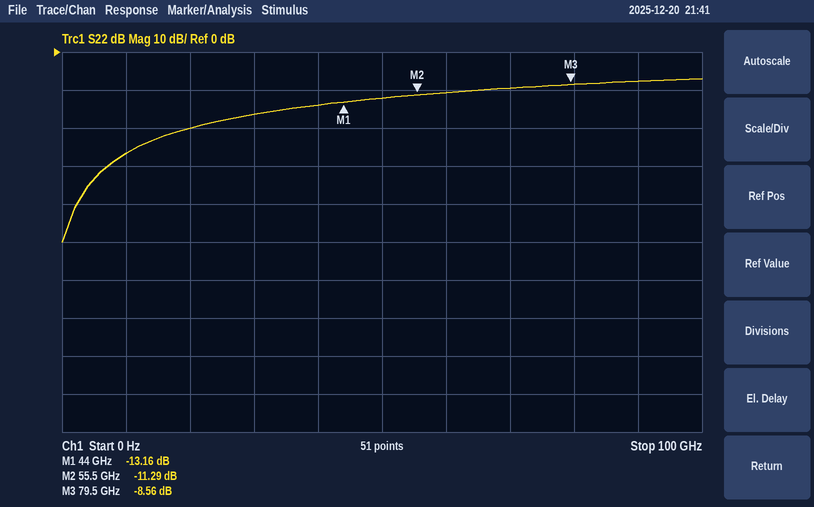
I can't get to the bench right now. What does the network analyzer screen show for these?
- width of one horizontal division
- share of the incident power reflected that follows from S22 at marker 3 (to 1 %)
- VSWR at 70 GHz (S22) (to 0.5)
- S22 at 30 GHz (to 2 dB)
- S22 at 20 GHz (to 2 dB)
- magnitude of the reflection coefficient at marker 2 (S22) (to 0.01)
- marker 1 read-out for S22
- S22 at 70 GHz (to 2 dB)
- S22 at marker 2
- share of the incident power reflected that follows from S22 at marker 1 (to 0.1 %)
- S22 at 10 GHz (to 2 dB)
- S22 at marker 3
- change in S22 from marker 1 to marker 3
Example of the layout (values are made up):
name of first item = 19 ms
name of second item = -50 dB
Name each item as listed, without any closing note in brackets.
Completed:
width of one horizontal division = 10 GHz
share of the incident power reflected that follows from S22 at marker 3 = 14 %
VSWR at 70 GHz (S22) = 2.0
S22 at 30 GHz = -16 dB
S22 at 20 GHz = -20 dB
magnitude of the reflection coefficient at marker 2 (S22) = 0.27
marker 1 read-out for S22 = -13.16 dB
S22 at 70 GHz = -10 dB
S22 at marker 2 = -11.29 dB
share of the incident power reflected that follows from S22 at marker 1 = 4.8 %
S22 at 10 GHz = -26 dB
S22 at marker 3 = -8.56 dB
change in S22 from marker 1 to marker 3 = 4.60 dB
